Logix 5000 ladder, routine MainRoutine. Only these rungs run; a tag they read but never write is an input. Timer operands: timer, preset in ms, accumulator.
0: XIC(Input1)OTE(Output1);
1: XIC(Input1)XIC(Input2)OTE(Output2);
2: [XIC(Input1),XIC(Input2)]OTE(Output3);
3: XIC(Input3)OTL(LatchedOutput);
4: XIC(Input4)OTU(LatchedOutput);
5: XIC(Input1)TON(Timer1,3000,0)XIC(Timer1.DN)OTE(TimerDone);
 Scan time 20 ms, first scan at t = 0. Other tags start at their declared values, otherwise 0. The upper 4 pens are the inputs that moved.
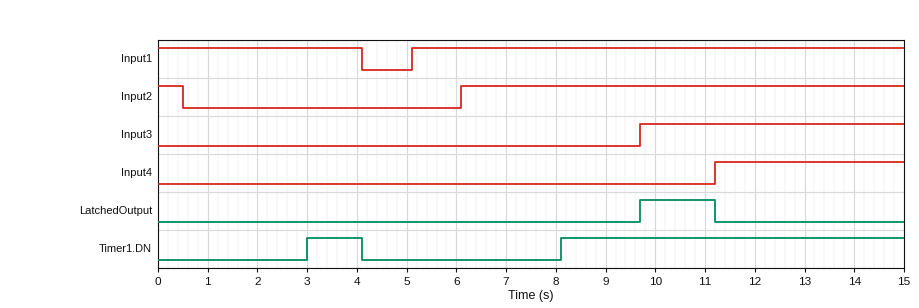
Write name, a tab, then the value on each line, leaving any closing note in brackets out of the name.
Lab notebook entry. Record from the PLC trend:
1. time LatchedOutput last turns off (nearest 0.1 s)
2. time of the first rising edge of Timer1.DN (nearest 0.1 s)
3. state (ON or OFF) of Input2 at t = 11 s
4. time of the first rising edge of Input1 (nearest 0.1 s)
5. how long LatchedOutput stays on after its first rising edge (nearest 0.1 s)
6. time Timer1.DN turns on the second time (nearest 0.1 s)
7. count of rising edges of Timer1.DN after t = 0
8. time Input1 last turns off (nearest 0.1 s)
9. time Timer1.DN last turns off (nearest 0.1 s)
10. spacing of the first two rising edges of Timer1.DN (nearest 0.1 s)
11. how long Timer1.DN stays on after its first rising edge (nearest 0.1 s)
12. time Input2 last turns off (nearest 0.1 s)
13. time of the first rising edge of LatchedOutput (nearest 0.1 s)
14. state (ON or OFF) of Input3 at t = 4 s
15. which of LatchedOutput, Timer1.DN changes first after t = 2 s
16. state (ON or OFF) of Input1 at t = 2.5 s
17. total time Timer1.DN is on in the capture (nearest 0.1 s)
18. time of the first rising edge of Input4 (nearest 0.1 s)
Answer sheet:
time LatchedOutput last turns off	11.2 s
time of the first rising edge of Timer1.DN	3.0 s
state (ON or OFF) of Input2 at t = 11 s	ON
time of the first rising edge of Input1	5.1 s
how long LatchedOutput stays on after its first rising edge	1.5 s
time Timer1.DN turns on the second time	8.1 s
count of rising edges of Timer1.DN after t = 0	2
time Input1 last turns off	4.1 s
time Timer1.DN last turns off	4.1 s
spacing of the first two rising edges of Timer1.DN	5.1 s
how long Timer1.DN stays on after its first rising edge	1.1 s
time Input2 last turns off	0.5 s
time of the first rising edge of LatchedOutput	9.7 s
state (ON or OFF) of Input3 at t = 4 s	OFF
which of LatchedOutput, Timer1.DN changes first after t = 2 s	Timer1.DN
state (ON or OFF) of Input1 at t = 2.5 s	ON
total time Timer1.DN is on in the capture	8.0 s
time of the first rising edge of Input4	11.2 s
